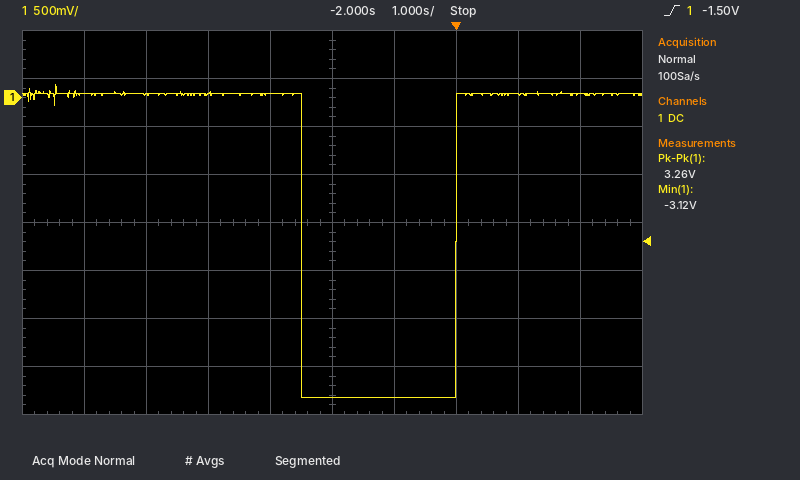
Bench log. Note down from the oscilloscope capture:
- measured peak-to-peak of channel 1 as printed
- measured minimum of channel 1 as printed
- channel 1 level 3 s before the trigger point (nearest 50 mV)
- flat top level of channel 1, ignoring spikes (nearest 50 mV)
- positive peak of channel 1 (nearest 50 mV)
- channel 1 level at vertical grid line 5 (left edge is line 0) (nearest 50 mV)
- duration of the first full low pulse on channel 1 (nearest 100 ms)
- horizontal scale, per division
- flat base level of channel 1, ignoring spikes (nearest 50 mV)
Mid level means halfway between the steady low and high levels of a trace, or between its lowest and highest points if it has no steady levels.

3.26 V
-3.12 V
50 mV
50 mV
150 mV
-3.10 V
2.5 s
1 s
-3.10 V
